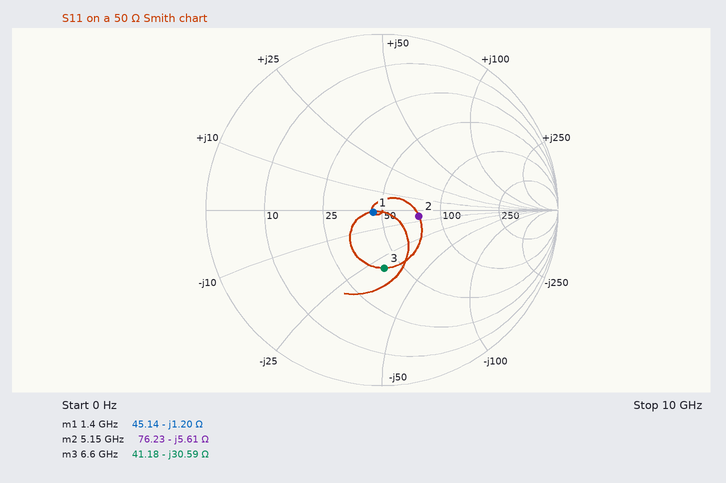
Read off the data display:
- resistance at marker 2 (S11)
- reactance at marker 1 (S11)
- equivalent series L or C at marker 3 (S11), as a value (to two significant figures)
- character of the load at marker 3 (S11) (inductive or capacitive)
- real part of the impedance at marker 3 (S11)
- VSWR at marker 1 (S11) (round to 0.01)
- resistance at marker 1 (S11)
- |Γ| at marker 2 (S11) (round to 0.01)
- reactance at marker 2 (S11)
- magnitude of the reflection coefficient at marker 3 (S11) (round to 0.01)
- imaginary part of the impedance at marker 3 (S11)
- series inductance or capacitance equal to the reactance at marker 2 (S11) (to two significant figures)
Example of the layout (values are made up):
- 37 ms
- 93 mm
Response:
- 76.23 Ω
- -1.20 Ω
- 790 fF
- capacitive
- 41.18 Ω
- 1.11
- 45.14 Ω
- 0.21
- -5.61 Ω
- 0.33
- -30.59 Ω
- 5.5 pF
